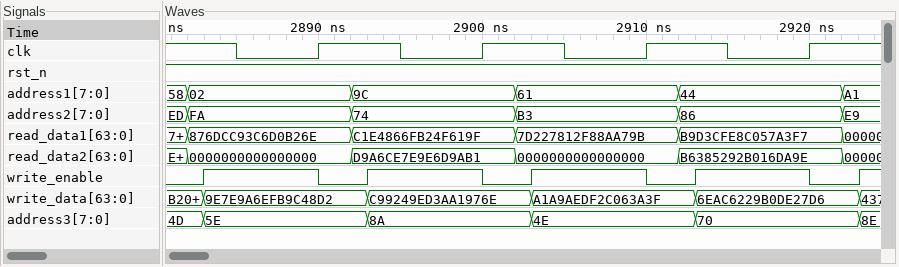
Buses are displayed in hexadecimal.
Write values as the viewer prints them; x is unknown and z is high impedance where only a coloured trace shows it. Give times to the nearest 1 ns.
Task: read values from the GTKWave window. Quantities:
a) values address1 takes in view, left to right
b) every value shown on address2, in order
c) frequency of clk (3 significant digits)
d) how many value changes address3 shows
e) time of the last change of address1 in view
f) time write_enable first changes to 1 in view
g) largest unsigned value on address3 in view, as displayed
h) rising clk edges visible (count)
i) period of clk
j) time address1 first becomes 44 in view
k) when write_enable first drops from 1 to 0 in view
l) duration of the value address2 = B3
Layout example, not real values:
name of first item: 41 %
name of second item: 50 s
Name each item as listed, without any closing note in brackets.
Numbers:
values address1 takes in view, left to right: 58, 02, 9C, 61, 44, A1
every value shown on address2, in order: ED, FA, 74, B3, 86, E9
frequency of clk: 100 MHz
how many value changes address3 shows: 5
time of the last change of address1 in view: 2922 ns
time write_enable first changes to 1 in view: 2883 ns
largest unsigned value on address3 in view, as displayed: 8E
rising clk edges visible: 4
period of clk: 10 ns
time address1 first becomes 44 in view: 2912 ns
when write_enable first drops from 1 to 0 in view: 2890 ns
duration of the value address2 = B3: 10 ns
